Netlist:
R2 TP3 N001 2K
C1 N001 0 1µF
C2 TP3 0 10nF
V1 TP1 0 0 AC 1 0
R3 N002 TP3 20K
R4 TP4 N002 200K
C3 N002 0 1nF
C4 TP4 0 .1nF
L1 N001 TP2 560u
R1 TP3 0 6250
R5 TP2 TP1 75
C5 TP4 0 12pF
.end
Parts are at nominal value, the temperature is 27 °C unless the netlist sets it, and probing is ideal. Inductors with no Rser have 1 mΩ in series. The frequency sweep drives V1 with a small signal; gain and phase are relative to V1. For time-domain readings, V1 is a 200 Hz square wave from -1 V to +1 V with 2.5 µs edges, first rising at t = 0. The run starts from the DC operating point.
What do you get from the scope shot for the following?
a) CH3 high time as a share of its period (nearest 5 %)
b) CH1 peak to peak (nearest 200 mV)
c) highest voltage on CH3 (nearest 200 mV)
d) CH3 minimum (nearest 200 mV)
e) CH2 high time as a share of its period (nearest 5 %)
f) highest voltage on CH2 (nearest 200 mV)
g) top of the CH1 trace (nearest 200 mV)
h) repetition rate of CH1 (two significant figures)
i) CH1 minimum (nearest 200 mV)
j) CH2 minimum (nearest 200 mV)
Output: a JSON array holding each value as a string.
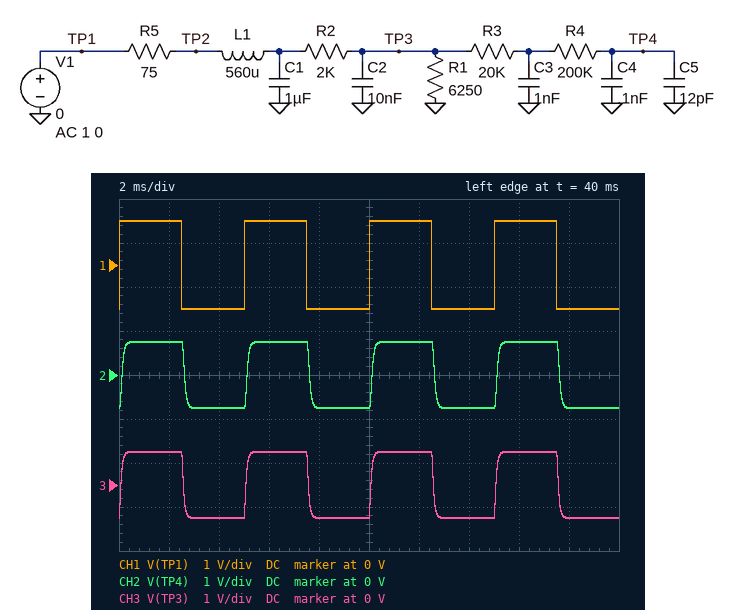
["50 %", "2.0 V", "800 mV", "-800 mV", "50 %", "800 mV", "1.0 V", "200 Hz", "-1.0 V", "-800 mV"]
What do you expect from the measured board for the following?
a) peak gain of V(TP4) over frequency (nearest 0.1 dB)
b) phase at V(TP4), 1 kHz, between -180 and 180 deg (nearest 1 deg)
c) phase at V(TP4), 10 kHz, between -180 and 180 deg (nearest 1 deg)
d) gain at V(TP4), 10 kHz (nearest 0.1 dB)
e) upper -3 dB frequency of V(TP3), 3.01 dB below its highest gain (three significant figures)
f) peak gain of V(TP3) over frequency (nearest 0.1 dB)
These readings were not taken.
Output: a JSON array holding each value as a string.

["-2.5 dB", "-48 deg", "107 deg", "-28.6 dB", "2.20 kHz", "-2.5 dB"]
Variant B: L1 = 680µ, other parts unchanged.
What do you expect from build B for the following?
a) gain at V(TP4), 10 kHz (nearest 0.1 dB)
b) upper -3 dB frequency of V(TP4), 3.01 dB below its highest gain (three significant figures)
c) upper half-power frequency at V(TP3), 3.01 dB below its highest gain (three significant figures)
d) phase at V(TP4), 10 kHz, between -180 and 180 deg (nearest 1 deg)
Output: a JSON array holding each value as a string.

["-28.9 dB", "1.92 kHz", "2.25 kHz", "102 deg"]
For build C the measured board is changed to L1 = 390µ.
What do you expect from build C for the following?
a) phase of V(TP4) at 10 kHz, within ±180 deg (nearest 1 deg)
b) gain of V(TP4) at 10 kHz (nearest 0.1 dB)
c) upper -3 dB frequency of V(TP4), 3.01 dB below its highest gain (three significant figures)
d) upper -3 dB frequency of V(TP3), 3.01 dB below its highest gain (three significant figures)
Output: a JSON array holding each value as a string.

["115 deg", "-28.4 dB", "1.85 kHz", "2.14 kHz"]
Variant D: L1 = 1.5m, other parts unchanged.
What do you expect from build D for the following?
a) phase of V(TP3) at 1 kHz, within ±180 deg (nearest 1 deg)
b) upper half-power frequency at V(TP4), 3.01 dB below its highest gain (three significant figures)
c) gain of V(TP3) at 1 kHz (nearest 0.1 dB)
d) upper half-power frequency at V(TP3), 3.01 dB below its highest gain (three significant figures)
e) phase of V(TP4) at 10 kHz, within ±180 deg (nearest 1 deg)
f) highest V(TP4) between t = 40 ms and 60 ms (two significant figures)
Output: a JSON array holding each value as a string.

["-33 deg", "2.15 kHz", "-3.0 dB", "2.56 kHz", "75 deg", "750 mV"]
